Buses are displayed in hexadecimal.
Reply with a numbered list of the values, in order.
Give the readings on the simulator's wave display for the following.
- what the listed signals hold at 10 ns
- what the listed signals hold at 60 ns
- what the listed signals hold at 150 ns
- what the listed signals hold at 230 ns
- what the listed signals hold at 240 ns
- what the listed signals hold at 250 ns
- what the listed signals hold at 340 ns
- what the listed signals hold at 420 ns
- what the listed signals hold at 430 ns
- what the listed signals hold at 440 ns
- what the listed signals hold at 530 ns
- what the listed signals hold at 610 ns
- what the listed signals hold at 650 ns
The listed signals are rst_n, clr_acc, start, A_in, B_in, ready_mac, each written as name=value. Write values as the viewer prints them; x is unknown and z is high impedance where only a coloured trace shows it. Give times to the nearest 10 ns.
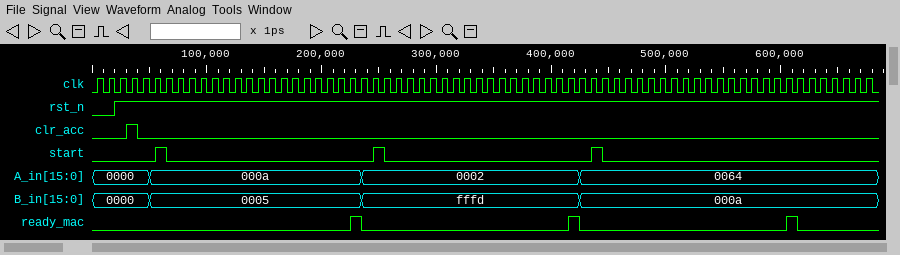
1. rst_n=0, clr_acc=0, start=0, A_in=0000, B_in=0000, ready_mac=0
2. rst_n=1, clr_acc=0, start=1, A_in=000a, B_in=0005, ready_mac=0
3. rst_n=1, clr_acc=0, start=0, A_in=000a, B_in=0005, ready_mac=0
4. rst_n=1, clr_acc=0, start=0, A_in=000a, B_in=0005, ready_mac=1
5. rst_n=1, clr_acc=0, start=0, A_in=0002, B_in=fffd, ready_mac=0
6. rst_n=1, clr_acc=0, start=1, A_in=0002, B_in=fffd, ready_mac=0
7. rst_n=1, clr_acc=0, start=0, A_in=0002, B_in=fffd, ready_mac=0
8. rst_n=1, clr_acc=0, start=0, A_in=0002, B_in=fffd, ready_mac=1
9. rst_n=1, clr_acc=0, start=0, A_in=0064, B_in=000a, ready_mac=0
10. rst_n=1, clr_acc=0, start=1, A_in=0064, B_in=000a, ready_mac=0
11. rst_n=1, clr_acc=0, start=0, A_in=0064, B_in=000a, ready_mac=0
12. rst_n=1, clr_acc=0, start=0, A_in=0064, B_in=000a, ready_mac=1
13. rst_n=1, clr_acc=0, start=0, A_in=0064, B_in=000a, ready_mac=0
